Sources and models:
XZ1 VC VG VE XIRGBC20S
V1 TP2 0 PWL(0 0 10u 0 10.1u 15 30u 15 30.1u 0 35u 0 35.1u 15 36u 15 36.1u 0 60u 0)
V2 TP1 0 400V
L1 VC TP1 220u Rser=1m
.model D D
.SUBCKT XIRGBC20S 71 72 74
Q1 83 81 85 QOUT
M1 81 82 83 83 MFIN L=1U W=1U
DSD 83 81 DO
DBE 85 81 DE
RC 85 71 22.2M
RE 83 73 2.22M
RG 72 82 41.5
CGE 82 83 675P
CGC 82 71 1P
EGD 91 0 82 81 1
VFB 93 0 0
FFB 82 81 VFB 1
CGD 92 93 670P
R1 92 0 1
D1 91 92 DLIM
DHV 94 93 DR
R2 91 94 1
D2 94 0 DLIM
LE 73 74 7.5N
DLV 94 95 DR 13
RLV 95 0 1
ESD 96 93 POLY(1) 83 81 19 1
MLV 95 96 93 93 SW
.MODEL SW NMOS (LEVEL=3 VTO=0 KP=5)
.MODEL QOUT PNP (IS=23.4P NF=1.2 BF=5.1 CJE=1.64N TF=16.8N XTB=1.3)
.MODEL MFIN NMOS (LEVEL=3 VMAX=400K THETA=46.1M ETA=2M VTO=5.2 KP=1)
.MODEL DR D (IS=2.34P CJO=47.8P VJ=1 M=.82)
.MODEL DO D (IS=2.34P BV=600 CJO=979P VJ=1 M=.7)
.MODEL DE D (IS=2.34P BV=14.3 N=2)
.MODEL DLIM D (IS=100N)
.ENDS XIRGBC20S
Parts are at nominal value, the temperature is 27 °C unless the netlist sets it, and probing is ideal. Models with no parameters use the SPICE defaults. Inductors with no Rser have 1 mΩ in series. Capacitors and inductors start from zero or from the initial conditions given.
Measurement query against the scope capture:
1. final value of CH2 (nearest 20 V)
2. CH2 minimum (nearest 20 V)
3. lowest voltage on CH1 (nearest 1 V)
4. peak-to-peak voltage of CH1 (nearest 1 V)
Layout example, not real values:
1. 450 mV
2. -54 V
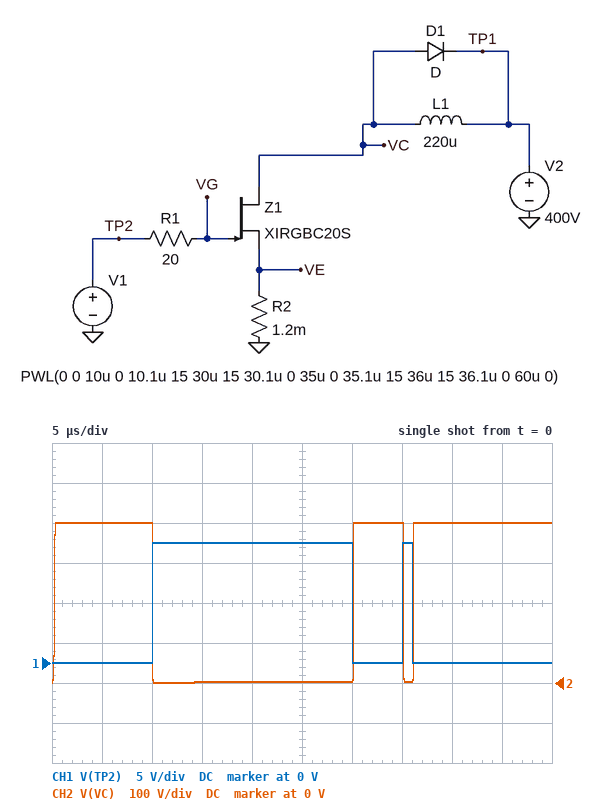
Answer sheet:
1. 400 V
2. 0 V
3. 0 V
4. 15 V
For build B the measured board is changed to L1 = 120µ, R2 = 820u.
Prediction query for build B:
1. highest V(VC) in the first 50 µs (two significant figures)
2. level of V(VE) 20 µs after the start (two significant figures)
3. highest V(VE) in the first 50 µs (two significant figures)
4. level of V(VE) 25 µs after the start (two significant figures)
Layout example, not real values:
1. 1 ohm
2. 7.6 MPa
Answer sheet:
1. 400 V
2. 27 mV
3. 57 mV
4. 41 mV
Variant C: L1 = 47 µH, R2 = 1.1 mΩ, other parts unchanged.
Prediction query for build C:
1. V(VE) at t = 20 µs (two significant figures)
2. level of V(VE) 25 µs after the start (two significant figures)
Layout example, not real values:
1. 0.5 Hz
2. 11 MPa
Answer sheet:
1. 93 mV
2. 130 mV
